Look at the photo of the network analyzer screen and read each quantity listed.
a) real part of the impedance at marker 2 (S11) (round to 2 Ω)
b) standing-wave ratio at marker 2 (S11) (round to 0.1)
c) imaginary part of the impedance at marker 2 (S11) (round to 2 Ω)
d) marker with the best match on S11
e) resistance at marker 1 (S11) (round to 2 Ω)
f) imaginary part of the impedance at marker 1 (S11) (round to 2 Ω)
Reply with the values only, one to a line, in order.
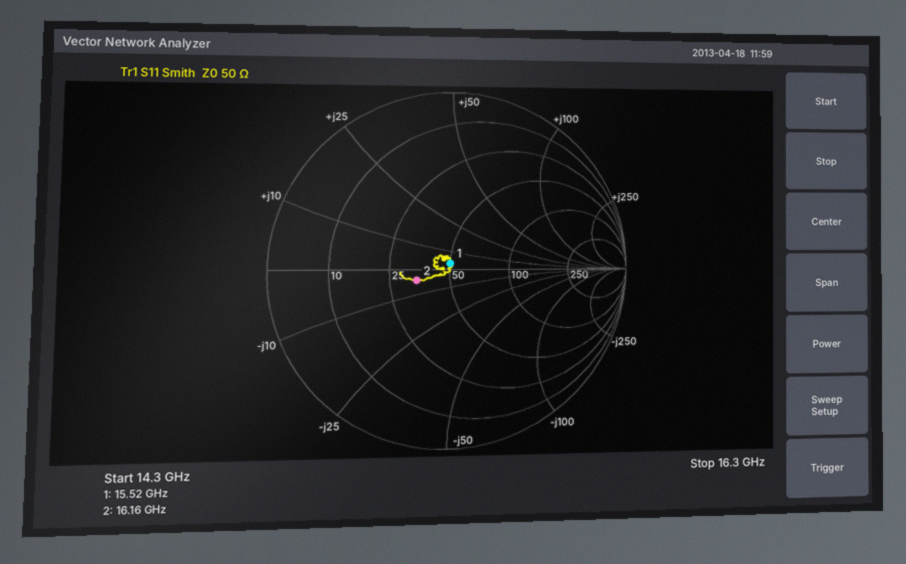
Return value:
34 Ω
1.5
-4 Ω
marker 1
50 Ω
+4 Ω
